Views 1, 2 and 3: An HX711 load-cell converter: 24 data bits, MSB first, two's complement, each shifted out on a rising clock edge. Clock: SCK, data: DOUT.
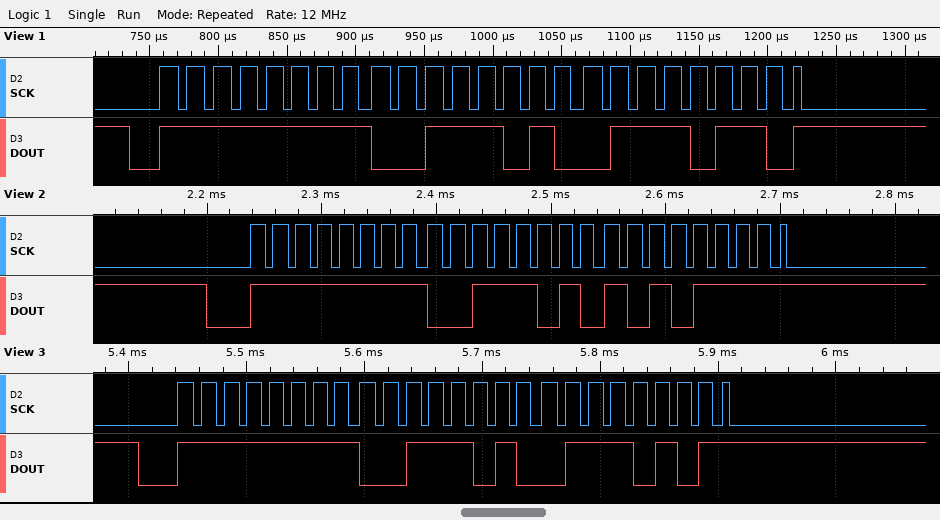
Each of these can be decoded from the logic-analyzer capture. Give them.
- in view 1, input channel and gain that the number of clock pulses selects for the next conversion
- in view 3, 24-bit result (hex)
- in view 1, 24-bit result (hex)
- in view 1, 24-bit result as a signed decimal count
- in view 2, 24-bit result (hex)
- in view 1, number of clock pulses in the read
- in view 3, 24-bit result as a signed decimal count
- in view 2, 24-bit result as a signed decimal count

channel A, gain 128
0xFF3A75
0xFF3A76
-50570
0xFF3AAF
25
-50571
-50513
